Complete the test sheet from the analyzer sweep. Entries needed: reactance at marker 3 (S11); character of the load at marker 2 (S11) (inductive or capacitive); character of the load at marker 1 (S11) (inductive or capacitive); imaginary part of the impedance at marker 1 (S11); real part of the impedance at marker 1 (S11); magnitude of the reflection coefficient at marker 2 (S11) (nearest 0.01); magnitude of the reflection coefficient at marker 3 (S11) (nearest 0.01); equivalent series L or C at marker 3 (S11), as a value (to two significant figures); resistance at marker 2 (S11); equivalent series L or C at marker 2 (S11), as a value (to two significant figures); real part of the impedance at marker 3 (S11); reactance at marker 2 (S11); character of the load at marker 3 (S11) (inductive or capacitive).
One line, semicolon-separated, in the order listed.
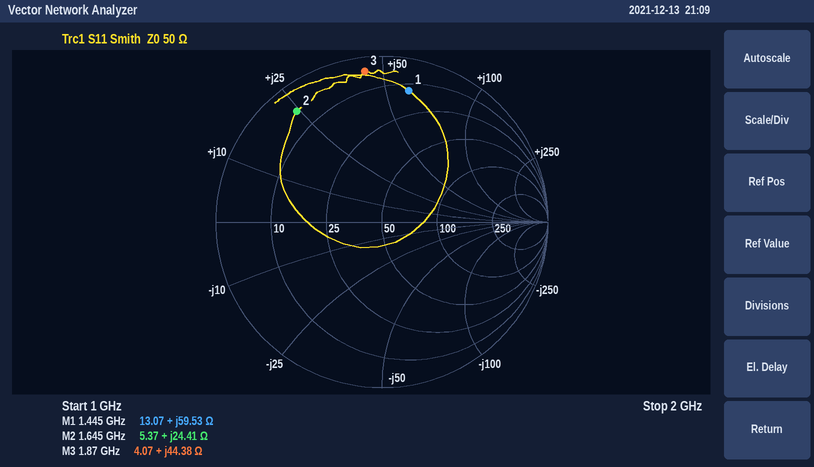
+44.38 Ω; inductive; inductive; +59.53 Ω; 13.07 Ω; 0.84; 0.91; 3.8 nH; 5.37 Ω; 2.4 nH; 4.07 Ω; +24.41 Ω; inductive
